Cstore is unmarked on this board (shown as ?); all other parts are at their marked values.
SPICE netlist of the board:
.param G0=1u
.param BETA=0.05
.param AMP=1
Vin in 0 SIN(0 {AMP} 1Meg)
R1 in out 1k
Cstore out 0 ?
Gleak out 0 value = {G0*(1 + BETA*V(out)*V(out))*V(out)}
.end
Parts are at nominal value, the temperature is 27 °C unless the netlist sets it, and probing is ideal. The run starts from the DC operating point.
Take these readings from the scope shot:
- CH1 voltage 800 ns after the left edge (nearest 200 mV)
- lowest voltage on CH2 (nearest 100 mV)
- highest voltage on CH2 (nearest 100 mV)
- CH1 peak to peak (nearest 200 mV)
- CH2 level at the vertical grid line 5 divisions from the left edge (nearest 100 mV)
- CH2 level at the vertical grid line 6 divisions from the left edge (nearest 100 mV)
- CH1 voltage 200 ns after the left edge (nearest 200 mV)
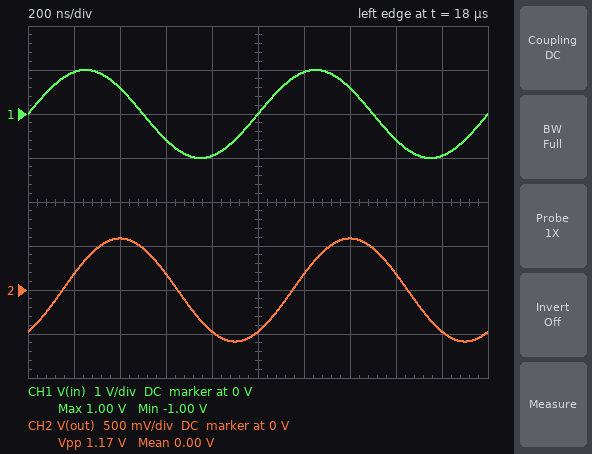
-1.0 V
-600 mV
600 mV
2.0 V
-500 mV
200 mV
1.0 V
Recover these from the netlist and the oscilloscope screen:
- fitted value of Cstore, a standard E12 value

220 pF
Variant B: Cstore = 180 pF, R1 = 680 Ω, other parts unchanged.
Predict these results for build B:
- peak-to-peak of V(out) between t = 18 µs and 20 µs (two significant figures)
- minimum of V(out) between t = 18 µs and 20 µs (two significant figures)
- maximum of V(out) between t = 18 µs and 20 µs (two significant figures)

1.6 V
-790 mV
790 mV
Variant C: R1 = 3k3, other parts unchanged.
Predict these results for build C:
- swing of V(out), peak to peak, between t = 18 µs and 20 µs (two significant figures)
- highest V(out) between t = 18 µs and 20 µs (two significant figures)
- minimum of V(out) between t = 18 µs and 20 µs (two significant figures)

430 mV
210 mV
-210 mV
